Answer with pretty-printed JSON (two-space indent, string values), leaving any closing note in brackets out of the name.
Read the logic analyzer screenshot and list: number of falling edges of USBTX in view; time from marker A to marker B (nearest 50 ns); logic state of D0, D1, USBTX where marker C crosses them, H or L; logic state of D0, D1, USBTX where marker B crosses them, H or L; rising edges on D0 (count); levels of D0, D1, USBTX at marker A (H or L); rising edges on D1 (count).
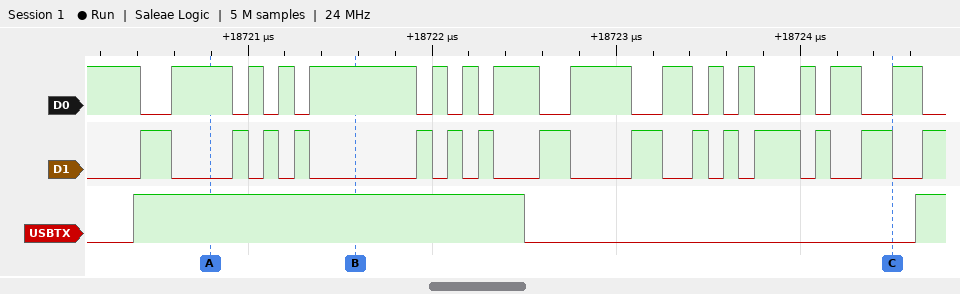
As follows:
{
  "number of falling edges of USBTX in view": "1",
  "time from marker A to marker B": "800 ns",
  "logic state of D0, D1, USBTX where marker C crosses them, H or L": "D0=H, D1=L, USBTX=L",
  "logic state of D0, D1, USBTX where marker B crosses them, H or L": "D0=H, D1=L, USBTX=H",
  "rising edges on D0": "14",
  "levels of D0, D1, USBTX at marker A": "D0=H, D1=L, USBTX=H",
  "rising edges on D1": "15"
}
